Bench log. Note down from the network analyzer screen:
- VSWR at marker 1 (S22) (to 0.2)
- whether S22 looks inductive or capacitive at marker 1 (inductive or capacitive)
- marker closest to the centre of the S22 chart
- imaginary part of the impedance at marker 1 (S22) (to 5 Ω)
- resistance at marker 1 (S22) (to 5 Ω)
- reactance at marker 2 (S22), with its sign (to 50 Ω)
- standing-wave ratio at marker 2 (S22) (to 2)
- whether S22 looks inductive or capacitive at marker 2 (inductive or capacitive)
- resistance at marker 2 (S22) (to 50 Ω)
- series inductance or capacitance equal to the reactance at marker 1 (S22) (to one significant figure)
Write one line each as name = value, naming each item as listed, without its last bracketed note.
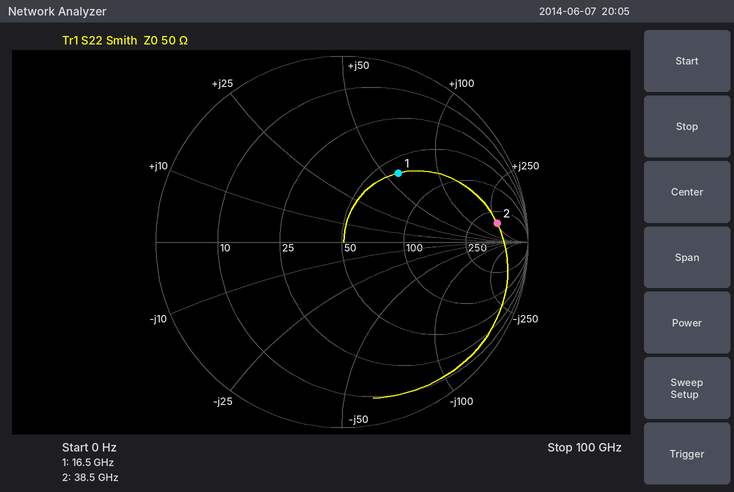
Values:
VSWR at marker 1 (S22) = 2.8
whether S22 looks inductive or capacitive at marker 1 = inductive
marker closest to the centre of the S22 chart = marker 1
imaginary part of the impedance at marker 1 (S22) = +60 Ω
resistance at marker 1 (S22) = 60 Ω
reactance at marker 2 (S22), with its sign = +250 Ω
standing-wave ratio at marker 2 (S22) = 12
whether S22 looks inductive or capacitive at marker 2 = inductive
resistance at marker 2 (S22) = 400 Ω
series inductance or capacitance equal to the reactance at marker 1 (S22) = 600 pH
